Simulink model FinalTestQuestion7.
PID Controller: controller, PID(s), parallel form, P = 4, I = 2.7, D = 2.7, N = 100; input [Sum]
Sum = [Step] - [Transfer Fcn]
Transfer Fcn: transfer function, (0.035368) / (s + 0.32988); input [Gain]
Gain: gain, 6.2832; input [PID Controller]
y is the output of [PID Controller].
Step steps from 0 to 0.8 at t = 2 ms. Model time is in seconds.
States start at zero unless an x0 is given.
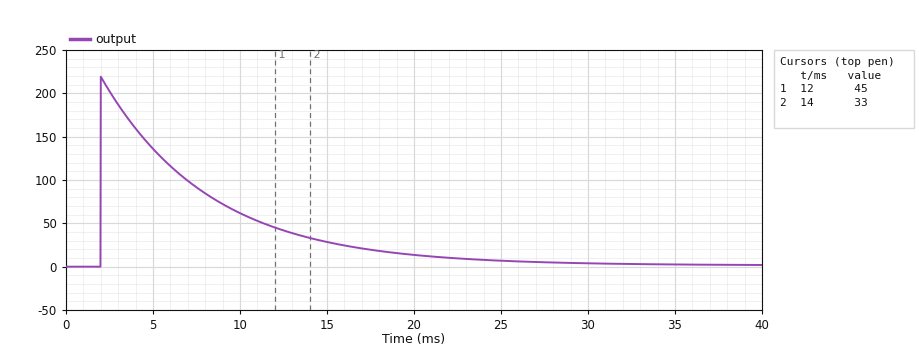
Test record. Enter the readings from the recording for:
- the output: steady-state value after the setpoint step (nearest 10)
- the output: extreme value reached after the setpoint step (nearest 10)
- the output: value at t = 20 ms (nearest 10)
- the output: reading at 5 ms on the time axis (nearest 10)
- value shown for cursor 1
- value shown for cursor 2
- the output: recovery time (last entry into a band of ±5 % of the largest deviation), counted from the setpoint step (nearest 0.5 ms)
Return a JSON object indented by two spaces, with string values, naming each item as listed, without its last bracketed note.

{
  "the output: steady-state value after the setpoint step": "0",
  "the output: extreme value reached after the setpoint step": "220",
  "the output: value at t = 20 ms": "10",
  "the output: reading at 5 ms on the time axis": "140",
  "value shown for cursor 1": "45",
  "value shown for cursor 2": "33",
  "the output: recovery time (last entry into a band of ±5 % of the largest deviation), counted from the setpoint step": "18.5 ms"
}
